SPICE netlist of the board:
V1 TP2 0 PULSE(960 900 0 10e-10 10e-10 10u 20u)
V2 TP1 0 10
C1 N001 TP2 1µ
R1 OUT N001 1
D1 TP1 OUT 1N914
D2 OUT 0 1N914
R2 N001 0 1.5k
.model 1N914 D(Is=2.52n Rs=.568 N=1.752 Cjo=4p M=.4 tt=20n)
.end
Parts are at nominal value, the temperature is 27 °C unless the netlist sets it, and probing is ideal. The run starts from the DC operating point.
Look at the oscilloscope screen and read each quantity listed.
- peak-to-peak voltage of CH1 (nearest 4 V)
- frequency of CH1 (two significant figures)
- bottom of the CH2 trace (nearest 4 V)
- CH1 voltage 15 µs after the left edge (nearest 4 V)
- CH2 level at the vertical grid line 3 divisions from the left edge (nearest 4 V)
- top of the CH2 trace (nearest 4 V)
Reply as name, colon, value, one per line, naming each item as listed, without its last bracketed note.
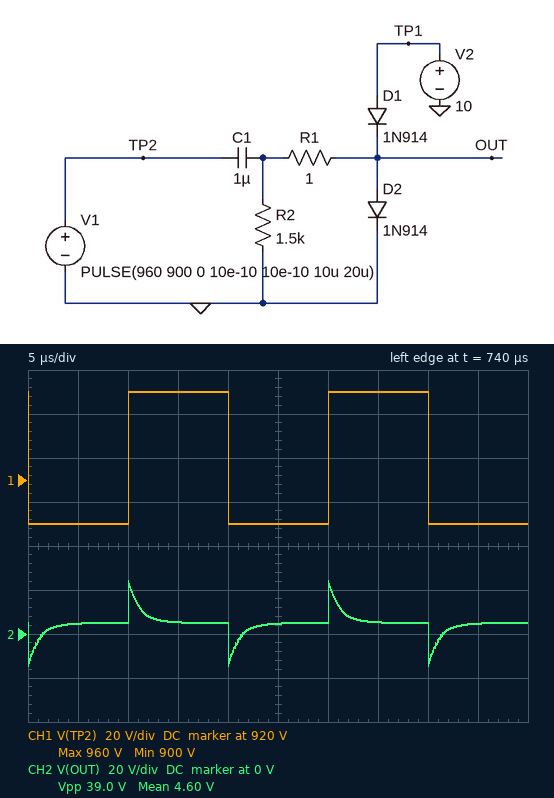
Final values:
peak-to-peak voltage of CH1: 60 V
frequency of CH1: 50 kHz
bottom of the CH2 trace: -16 V
CH1 voltage 15 µs after the left edge: 960 V
CH2 level at the vertical grid line 3 divisions from the left edge: 4 V
top of the CH2 trace: 24 V
